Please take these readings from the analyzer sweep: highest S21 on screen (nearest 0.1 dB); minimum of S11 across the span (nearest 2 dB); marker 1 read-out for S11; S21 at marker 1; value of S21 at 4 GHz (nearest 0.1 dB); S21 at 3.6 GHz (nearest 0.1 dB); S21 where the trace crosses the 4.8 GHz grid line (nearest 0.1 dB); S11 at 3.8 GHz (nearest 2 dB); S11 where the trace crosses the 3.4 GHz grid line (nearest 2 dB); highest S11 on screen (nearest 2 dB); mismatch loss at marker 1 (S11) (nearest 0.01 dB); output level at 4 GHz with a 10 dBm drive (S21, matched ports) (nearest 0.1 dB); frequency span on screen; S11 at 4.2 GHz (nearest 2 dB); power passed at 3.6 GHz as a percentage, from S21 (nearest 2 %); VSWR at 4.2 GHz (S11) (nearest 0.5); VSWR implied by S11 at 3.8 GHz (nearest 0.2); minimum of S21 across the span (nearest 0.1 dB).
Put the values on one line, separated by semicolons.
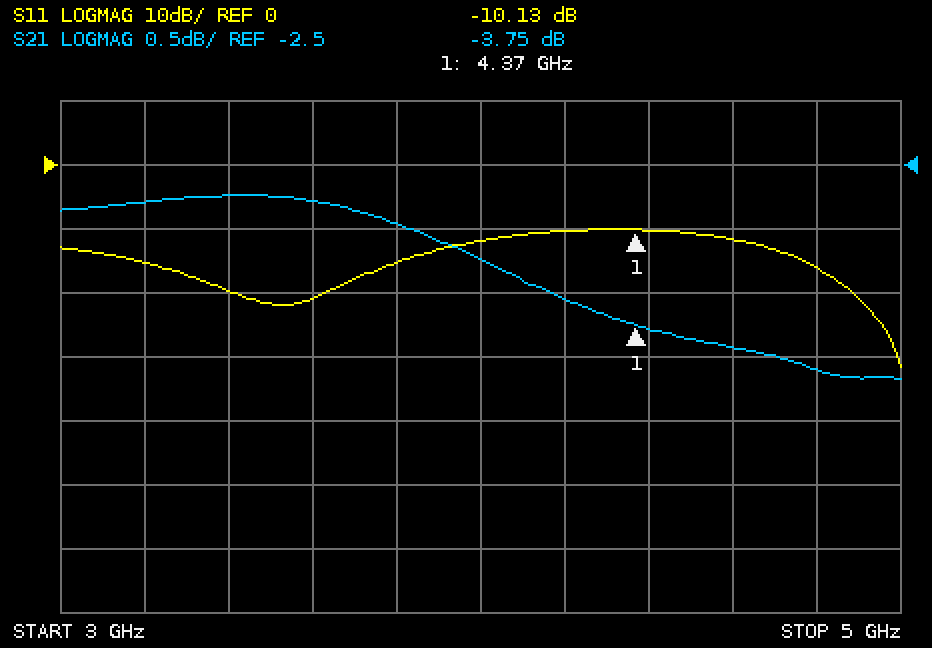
-2.7 dB; -32 dB; -10.13 dB; -3.75 dB; -3.2 dB; -2.8 dB; -4.1 dB; -16 dB; -20 dB; -10 dB; 0.44 dB; 6.8 dBm; 2 GHz; -10 dB; 52 %; 2.0; 1.4; -4.2 dB
